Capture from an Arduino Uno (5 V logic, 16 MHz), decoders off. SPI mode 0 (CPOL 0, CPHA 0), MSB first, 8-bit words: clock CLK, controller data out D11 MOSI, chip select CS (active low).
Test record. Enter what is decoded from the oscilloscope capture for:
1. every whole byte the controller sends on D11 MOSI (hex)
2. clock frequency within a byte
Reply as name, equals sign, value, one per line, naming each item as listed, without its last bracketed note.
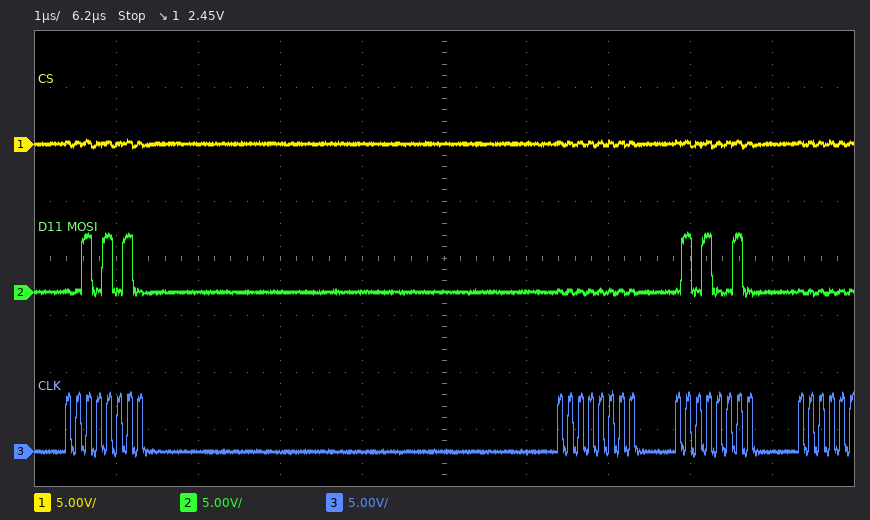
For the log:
every whole byte the controller sends on D11 MOSI = 2A 00 52
clock frequency within a byte = 8 MHz
